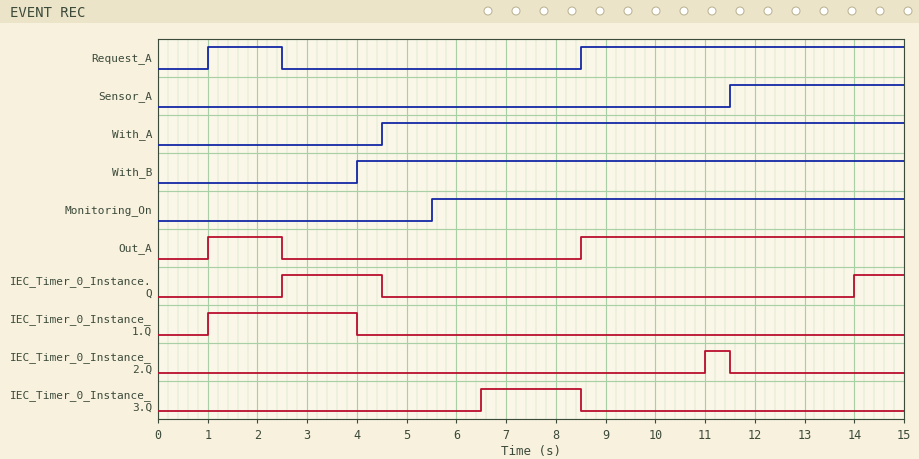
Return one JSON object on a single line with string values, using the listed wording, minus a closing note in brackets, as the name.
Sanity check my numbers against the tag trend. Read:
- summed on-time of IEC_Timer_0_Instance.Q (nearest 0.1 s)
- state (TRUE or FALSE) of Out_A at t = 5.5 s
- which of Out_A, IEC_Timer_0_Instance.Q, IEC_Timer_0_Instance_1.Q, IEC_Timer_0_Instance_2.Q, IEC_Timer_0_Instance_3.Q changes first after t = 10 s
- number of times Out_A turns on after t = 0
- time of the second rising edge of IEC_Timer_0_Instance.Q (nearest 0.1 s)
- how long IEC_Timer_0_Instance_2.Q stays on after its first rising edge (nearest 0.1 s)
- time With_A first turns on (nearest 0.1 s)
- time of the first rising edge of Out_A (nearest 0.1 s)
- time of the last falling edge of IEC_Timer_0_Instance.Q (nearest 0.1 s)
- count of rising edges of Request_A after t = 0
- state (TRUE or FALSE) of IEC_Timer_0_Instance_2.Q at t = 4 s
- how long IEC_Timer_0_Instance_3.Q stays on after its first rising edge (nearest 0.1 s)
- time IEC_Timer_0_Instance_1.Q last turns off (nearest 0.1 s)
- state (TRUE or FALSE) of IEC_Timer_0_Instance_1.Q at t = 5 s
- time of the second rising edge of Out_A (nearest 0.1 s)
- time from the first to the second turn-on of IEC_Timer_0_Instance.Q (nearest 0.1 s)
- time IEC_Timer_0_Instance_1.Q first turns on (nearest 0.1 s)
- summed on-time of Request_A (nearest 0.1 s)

{"summed on-time of IEC_Timer_0_Instance.Q": "3.0 s", "state (TRUE or FALSE) of Out_A at t = 5.5 s": "FALSE", "which of Out_A, IEC_Timer_0_Instance.Q, IEC_Timer_0_Instance_1.Q, IEC_Timer_0_Instance_2.Q, IEC_Timer_0_Instance_3.Q changes first after t = 10 s": "IEC_Timer_0_Instance_2.Q", "number of times Out_A turns on after t = 0": "2", "time of the second rising edge of IEC_Timer_0_Instance.Q": "14.0 s", "how long IEC_Timer_0_Instance_2.Q stays on after its first rising edge": "0.5 s", "time With_A first turns on": "4.5 s", "time of the first rising edge of Out_A": "1.0 s", "time of the last falling edge of IEC_Timer_0_Instance.Q": "4.5 s", "count of rising edges of Request_A after t = 0": "2", "state (TRUE or FALSE) of IEC_Timer_0_Instance_2.Q at t = 4 s": "FALSE", "how long IEC_Timer_0_Instance_3.Q stays on after its first rising edge": "2.0 s", "time IEC_Timer_0_Instance_1.Q last turns off": "4.0 s", "state (TRUE or FALSE) of IEC_Timer_0_Instance_1.Q at t = 5 s": "FALSE", "time of the second rising edge of Out_A": "8.5 s", "time from the first to the second turn-on of IEC_Timer_0_Instance.Q": "11.5 s", "time IEC_Timer_0_Instance_1.Q first turns on": "1.0 s", "summed on-time of Request_A": "8.0 s"}
